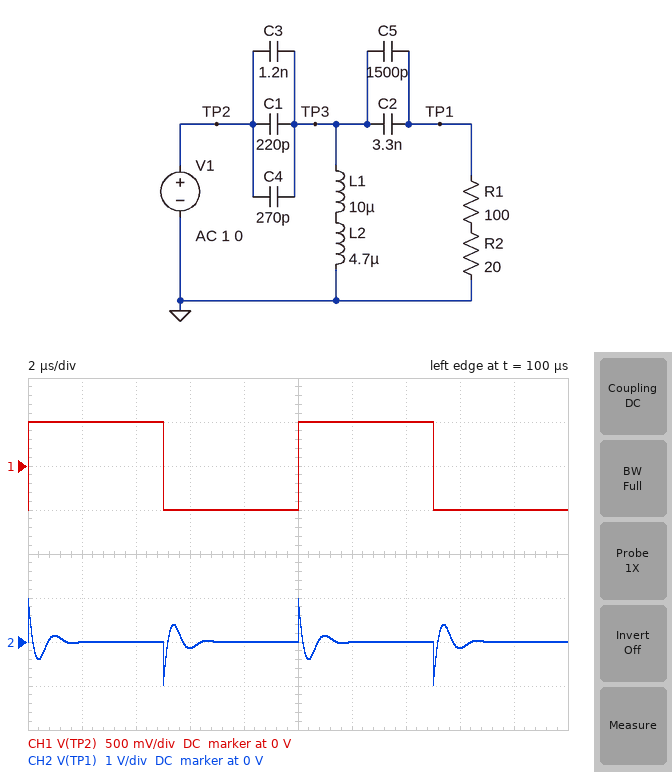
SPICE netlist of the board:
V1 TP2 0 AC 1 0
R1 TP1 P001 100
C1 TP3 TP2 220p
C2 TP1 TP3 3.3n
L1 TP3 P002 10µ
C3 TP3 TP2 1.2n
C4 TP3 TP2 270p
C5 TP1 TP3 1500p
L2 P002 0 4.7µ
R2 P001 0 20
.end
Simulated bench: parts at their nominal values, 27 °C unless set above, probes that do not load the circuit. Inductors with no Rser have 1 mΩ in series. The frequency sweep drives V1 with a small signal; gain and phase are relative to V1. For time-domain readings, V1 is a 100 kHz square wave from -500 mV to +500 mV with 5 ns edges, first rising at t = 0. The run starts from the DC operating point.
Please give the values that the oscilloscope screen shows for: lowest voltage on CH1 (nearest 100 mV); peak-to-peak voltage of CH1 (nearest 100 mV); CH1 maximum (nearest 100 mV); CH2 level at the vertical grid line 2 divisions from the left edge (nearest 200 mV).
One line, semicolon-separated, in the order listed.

-500 mV; 1.0 V; 500 mV; 0 V
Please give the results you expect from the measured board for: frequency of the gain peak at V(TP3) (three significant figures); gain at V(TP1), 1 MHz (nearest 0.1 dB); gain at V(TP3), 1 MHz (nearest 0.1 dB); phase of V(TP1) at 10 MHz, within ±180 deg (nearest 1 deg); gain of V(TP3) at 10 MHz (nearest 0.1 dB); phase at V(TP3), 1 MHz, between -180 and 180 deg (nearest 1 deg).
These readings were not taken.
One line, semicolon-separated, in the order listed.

1.07 MHz; 2.2 dB; 2.5 dB; 6 deg; 0 dB; 76 deg
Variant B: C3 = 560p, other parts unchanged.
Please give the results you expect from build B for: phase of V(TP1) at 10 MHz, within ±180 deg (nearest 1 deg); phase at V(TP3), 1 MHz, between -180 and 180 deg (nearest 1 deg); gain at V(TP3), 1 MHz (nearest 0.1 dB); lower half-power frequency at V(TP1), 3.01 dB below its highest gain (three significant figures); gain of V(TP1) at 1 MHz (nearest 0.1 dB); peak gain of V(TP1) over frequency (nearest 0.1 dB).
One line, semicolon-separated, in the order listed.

9 deg; 105 deg; -1.7 dB; 979 kHz; -2.0 dB; 0.7 dB
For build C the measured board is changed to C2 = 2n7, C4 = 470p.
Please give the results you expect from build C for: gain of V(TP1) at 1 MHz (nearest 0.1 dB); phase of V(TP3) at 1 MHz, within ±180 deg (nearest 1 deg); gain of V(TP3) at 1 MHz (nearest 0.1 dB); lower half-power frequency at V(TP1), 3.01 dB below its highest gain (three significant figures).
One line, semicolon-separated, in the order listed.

2.7 dB; 66 deg; 3.1 dB; 706 kHz
